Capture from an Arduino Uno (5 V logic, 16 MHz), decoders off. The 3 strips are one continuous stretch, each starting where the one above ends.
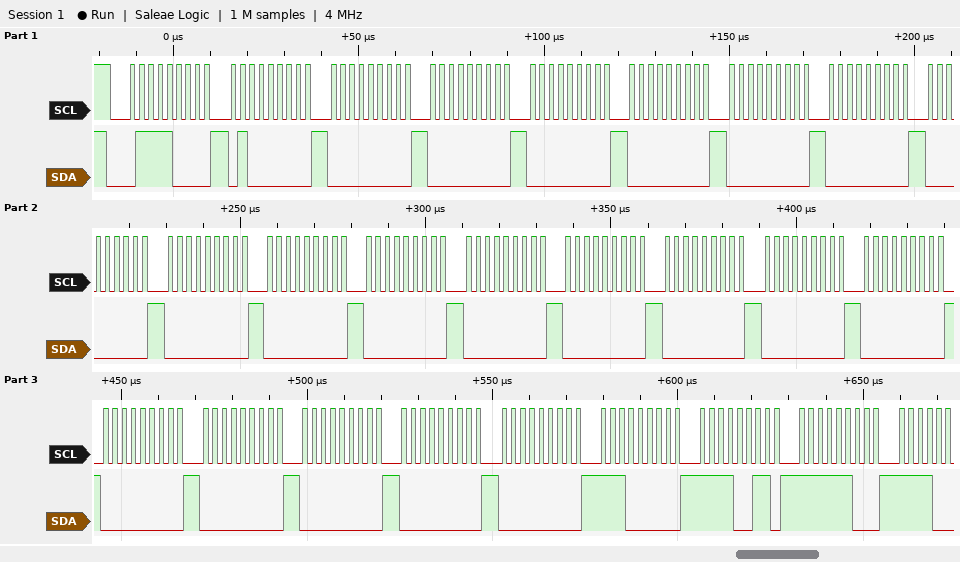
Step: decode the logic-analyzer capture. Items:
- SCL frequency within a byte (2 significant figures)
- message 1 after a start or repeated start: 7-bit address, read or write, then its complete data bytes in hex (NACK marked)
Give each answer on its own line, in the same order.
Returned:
400 kHz
0x3C write: 40 00 00 00 00 00 00 00 00 00 00 00 00 00 00 00 00 00 00 00 00 E0 F3 FC
